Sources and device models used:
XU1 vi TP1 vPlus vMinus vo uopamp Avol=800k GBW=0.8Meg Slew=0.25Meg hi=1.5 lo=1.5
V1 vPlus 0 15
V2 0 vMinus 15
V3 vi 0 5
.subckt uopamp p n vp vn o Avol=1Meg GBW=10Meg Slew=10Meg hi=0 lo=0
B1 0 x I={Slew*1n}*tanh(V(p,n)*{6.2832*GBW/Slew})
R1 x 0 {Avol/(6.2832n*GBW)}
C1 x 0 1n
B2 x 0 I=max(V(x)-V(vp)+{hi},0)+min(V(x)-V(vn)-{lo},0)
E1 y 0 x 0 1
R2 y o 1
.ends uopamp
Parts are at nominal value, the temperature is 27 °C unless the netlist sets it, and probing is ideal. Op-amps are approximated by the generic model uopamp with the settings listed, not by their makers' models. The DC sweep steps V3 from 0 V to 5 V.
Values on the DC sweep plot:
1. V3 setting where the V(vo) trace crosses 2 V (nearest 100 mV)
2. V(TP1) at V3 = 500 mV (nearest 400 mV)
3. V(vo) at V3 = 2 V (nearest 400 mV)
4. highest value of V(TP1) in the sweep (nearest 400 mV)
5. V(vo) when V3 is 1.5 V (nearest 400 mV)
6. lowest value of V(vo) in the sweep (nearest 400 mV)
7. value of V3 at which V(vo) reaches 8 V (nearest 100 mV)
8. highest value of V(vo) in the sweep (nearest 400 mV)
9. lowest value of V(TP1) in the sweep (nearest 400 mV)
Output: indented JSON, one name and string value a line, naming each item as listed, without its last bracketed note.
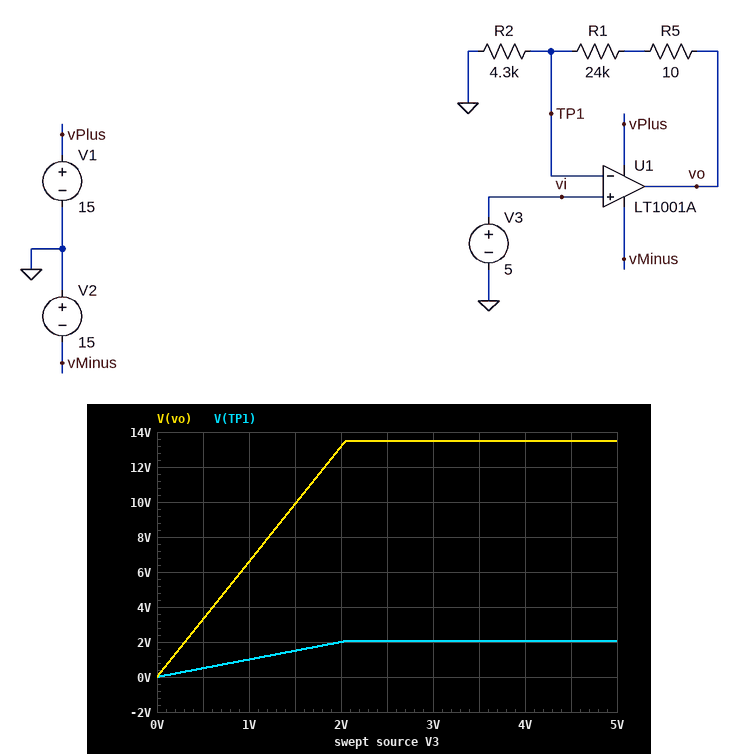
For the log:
{
  "V3 setting where the V(vo) trace crosses 2 V": "300 mV",
  "V(TP1) at V3 = 500 mV": "400 mV",
  "V(vo) at V3 = 2 V": "13.2 V",
  "highest value of V(TP1) in the sweep": "2.0 V",
  "V(vo) when V3 is 1.5 V": "10.0 V",
  "lowest value of V(vo) in the sweep": "0 V",
  "value of V3 at which V(vo) reaches 8 V": "1.2 V",
  "highest value of V(vo) in the sweep": "13.6 V",
  "lowest value of V(TP1) in the sweep": "0 V"
}
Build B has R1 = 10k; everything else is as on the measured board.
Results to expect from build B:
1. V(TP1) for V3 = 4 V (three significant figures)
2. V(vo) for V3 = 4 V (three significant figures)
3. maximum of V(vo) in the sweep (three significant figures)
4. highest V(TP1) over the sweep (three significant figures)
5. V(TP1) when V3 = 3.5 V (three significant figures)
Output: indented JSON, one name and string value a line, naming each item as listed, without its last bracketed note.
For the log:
{
  "V(TP1) for V3 = 4 V": "4.00 V",
  "V(vo) for V3 = 4 V": "13.3 V",
  "maximum of V(vo) in the sweep": "13.5 V",
  "highest V(TP1) over the sweep": "4.06 V",
  "V(TP1) when V3 = 3.5 V": "3.50 V"
}
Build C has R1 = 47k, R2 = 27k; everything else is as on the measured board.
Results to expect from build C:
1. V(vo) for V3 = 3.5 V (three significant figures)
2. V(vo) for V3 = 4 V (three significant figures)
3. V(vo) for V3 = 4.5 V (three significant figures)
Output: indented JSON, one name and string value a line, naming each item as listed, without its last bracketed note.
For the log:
{
  "V(vo) for V3 = 3.5 V": "9.59 V",
  "V(vo) for V3 = 4 V": "11.0 V",
  "V(vo) for V3 = 4.5 V": "12.3 V"
}
